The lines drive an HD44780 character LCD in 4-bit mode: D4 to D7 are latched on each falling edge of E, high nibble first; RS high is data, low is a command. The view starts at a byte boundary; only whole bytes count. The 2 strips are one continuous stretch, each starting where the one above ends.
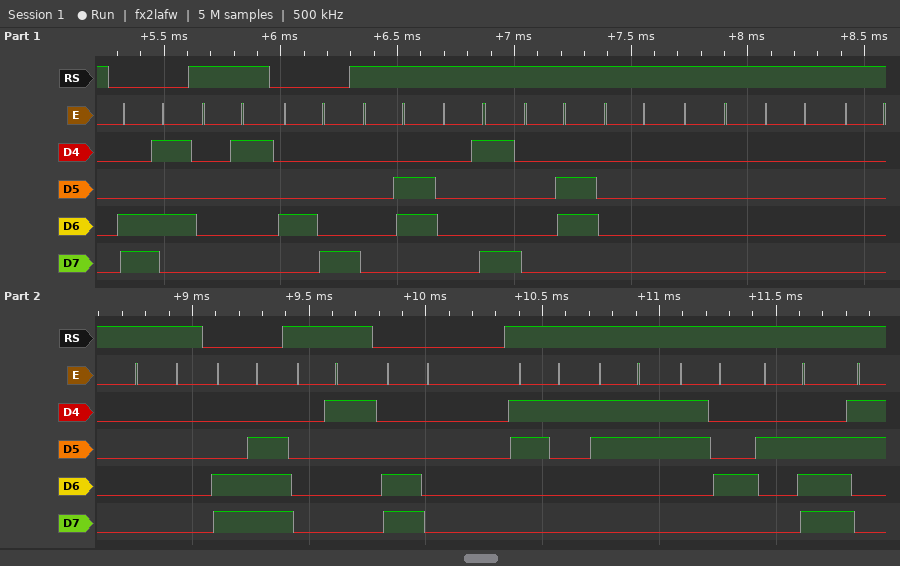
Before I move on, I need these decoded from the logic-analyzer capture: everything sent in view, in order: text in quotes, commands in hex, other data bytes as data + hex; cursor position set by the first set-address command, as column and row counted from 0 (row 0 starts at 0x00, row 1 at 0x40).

0xC5 data 01 0x48 data 06 09 06 00 00 00 00 00 0xCE data 01 0xC0 "134."
column 5, row 1
